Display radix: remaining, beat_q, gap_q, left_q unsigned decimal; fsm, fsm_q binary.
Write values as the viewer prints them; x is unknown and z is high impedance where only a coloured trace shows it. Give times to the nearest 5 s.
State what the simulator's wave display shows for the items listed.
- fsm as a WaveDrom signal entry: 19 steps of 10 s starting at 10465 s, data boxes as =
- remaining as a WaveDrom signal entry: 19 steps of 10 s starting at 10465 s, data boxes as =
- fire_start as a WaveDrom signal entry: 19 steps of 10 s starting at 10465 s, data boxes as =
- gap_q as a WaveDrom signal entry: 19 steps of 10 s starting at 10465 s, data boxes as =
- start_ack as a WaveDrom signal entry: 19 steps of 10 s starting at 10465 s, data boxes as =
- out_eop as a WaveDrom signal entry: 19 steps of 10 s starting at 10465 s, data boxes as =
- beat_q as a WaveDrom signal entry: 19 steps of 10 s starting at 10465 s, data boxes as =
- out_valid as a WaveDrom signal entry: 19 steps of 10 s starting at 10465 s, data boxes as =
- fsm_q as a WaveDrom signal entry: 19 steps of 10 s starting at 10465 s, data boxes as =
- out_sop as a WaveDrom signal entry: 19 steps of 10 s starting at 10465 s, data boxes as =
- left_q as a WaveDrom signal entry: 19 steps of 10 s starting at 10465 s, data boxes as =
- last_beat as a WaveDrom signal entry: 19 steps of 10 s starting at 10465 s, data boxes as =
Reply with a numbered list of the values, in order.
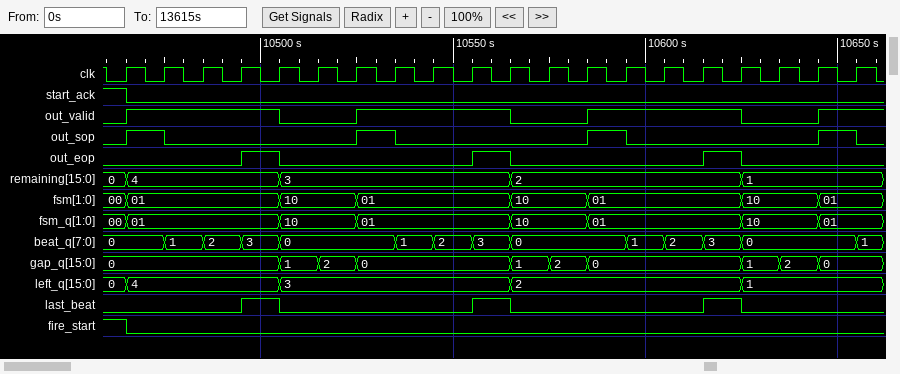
1. {name: 'fsm', wave: '=...=.=...=.=...=.=', data: '01 10 01 10 01 10 01'}
2. {name: 'remaining', wave: '=...=.....=.....=..', data: '4 3 2 1'}
3. {name: 'fire_start', wave: '0..................'}
4. {name: 'gap_q', wave: '=...===...===...===', data: '0 1 2 0 1 2 0 1 2 0'}
5. {name: 'start_ack', wave: '0..................'}
6. {name: 'out_eop', wave: '0..10....10....10..'}
7. {name: 'beat_q', wave: '=====..====..====..', data: '0 1 2 3 0 1 2 3 0 1 2 3 0'}
8. {name: 'out_valid', wave: '1...0.1...0.1...0.1'}
9. {name: 'fsm_q', wave: '=...=.=...=.=...=.=', data: '01 10 01 10 01 10 01'}
10. {name: 'out_sop', wave: '10....10....10....1'}
11. {name: 'left_q', wave: '=...=.....=.....=..', data: '4 3 2 1'}
12. {name: 'last_beat', wave: '0..10....10....10..'}
